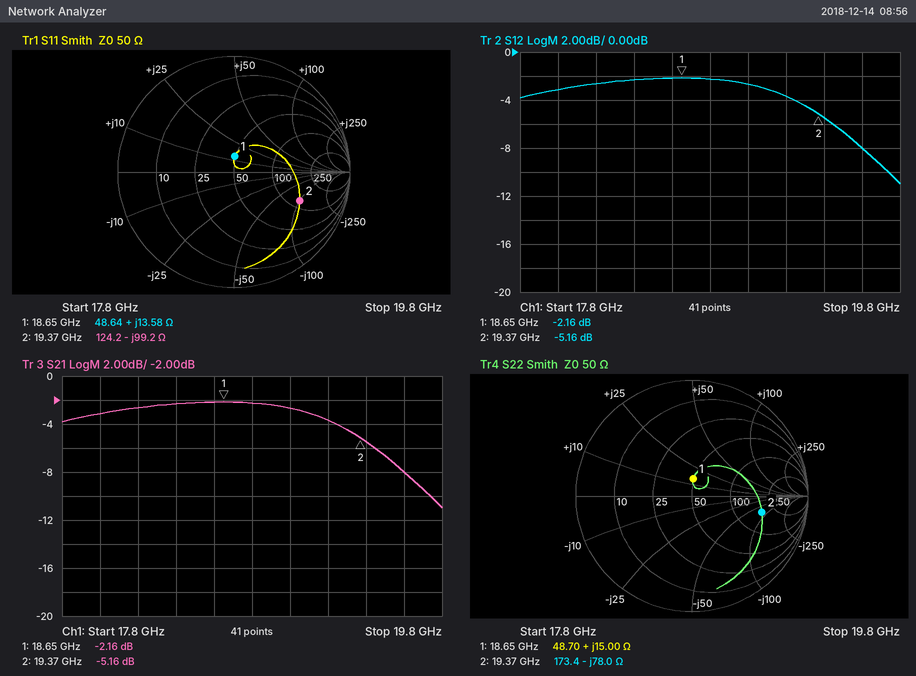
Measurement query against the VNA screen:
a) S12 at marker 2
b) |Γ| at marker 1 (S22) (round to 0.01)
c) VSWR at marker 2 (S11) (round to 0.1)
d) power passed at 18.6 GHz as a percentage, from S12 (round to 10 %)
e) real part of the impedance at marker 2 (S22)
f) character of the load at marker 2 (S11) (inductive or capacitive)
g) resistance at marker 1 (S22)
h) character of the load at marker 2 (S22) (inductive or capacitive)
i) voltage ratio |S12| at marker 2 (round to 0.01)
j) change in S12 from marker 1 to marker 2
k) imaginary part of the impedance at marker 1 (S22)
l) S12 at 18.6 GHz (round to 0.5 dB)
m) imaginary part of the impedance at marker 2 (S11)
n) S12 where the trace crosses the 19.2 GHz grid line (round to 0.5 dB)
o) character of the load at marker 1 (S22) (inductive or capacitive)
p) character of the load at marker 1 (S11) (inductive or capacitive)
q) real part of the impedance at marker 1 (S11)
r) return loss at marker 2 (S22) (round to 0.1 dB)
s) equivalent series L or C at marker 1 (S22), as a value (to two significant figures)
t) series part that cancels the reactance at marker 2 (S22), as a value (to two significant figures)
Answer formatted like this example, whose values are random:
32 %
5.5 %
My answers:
-5.16 dB
0.15
4.2
60 %
173.4 Ω
capacitive
48.70 Ω
capacitive
0.55
-3.00 dB
+15.00 Ω
-2.0 dB
-99.2 Ω
-3.5 dB
inductive
inductive
48.64 Ω
4.2 dB
130 pH
640 pH
